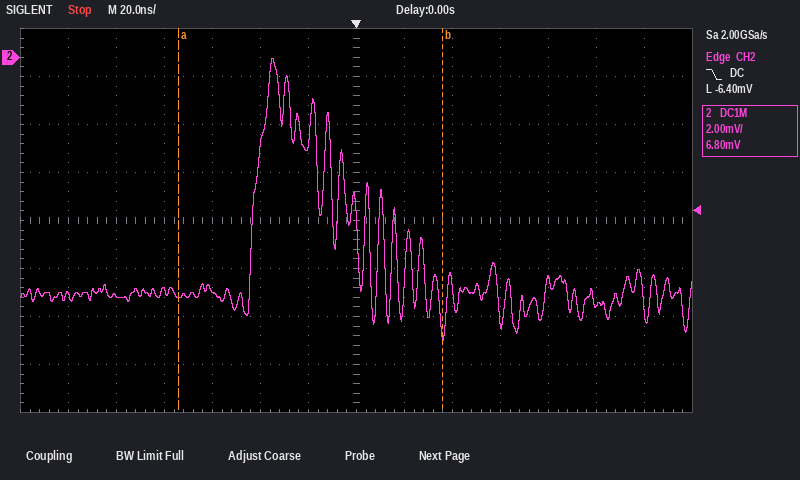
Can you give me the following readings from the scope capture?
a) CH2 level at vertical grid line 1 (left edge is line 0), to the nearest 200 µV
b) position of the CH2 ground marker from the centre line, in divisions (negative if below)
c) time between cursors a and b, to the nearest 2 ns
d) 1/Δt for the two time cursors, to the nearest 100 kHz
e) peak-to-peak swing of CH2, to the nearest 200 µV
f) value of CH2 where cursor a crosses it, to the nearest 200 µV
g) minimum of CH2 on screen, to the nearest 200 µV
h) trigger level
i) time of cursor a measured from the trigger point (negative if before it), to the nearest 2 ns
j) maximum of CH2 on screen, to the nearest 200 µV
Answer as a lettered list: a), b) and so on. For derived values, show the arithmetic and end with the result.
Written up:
a) -10.0 mV
b) +3.4 div
c) 110 ns
d) 1 / 110 ns ≈ 9.1 MHz
e) 0.0 mV − (-11.8 mV) = 11.8 mV
f) -10.0 mV
g) -11.8 mV
h) -6.40 mV
i) -74 ns
j) 0.0 mV
